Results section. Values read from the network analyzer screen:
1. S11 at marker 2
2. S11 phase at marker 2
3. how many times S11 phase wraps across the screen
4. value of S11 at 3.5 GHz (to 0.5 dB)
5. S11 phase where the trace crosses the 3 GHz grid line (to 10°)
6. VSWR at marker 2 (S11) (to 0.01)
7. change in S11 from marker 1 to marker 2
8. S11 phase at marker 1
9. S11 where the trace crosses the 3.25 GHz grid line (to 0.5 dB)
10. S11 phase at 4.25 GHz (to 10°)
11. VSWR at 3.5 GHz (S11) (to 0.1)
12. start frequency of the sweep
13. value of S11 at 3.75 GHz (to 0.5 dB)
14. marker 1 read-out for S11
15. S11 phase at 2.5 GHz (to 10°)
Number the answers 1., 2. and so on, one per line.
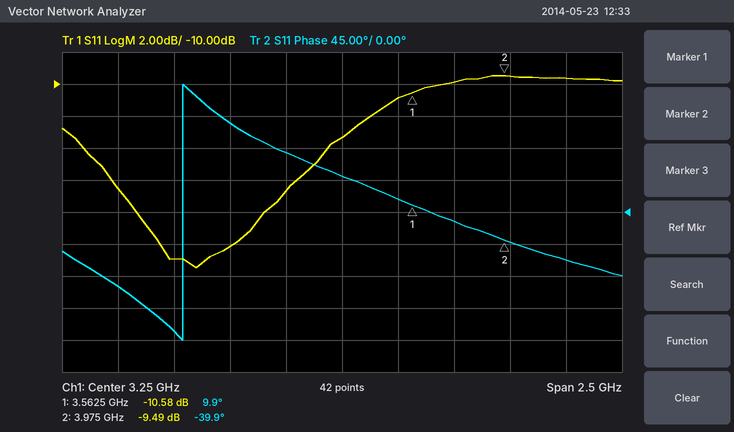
1. -9.49 dB
2. -39.9°
3. 1
4. -11.0 dB
5. 80°
6. 2.01
7. 1.09 dB
8. 9.9°
9. -13.5 dB
10. -70°
11. 1.8
12. 2 GHz
13. -10.0 dB
14. -10.58 dB
15. -170°
